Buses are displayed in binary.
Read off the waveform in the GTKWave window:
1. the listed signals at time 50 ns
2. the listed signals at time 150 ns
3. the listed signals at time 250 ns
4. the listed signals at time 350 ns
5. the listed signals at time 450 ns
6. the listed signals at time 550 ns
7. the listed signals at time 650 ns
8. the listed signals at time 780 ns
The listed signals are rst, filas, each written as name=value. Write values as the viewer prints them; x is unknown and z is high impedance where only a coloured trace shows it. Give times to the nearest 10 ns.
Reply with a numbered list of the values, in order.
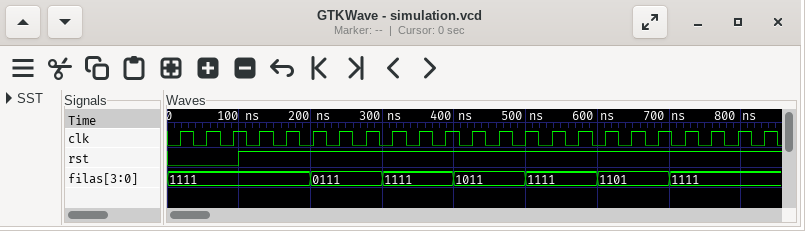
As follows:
1. rst=0, filas=1111
2. rst=1, filas=1111
3. rst=1, filas=0111
4. rst=1, filas=1111
5. rst=1, filas=1011
6. rst=1, filas=1111
7. rst=1, filas=1101
8. rst=1, filas=1111
